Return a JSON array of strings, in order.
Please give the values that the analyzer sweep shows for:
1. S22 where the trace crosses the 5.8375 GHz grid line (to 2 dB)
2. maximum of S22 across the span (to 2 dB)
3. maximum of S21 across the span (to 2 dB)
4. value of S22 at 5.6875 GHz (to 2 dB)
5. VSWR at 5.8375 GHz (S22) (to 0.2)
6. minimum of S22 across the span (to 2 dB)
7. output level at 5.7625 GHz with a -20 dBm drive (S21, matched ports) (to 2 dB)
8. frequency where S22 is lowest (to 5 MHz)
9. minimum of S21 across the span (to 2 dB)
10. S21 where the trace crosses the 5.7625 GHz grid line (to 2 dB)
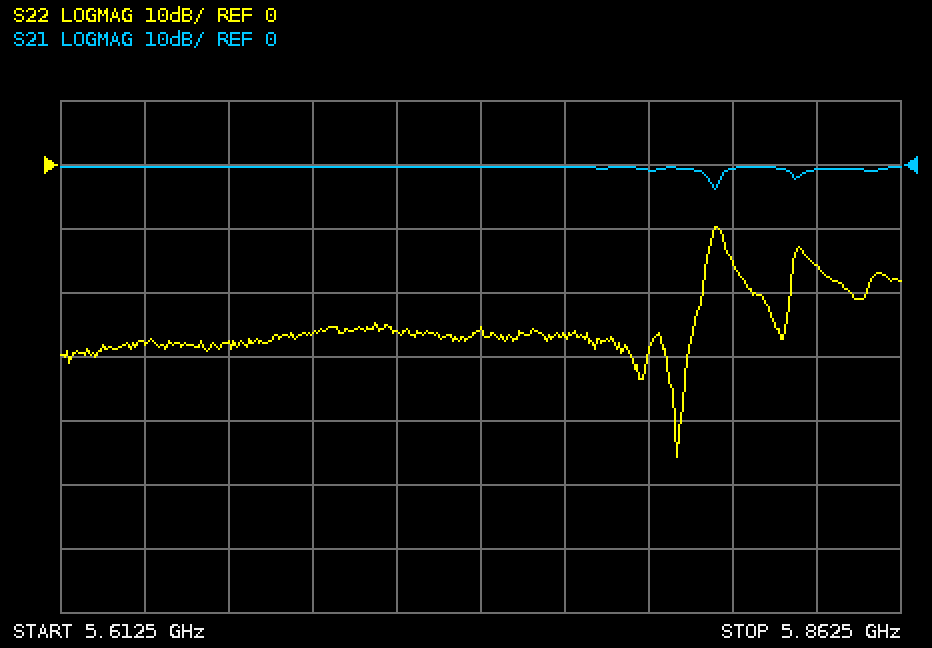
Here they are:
["-16 dB", "-10 dB", "0 dB", "-26 dB", "1.4", "-46 dB", "-20 dBm", "5.795 GHz", "-4 dB", "0 dB"]
